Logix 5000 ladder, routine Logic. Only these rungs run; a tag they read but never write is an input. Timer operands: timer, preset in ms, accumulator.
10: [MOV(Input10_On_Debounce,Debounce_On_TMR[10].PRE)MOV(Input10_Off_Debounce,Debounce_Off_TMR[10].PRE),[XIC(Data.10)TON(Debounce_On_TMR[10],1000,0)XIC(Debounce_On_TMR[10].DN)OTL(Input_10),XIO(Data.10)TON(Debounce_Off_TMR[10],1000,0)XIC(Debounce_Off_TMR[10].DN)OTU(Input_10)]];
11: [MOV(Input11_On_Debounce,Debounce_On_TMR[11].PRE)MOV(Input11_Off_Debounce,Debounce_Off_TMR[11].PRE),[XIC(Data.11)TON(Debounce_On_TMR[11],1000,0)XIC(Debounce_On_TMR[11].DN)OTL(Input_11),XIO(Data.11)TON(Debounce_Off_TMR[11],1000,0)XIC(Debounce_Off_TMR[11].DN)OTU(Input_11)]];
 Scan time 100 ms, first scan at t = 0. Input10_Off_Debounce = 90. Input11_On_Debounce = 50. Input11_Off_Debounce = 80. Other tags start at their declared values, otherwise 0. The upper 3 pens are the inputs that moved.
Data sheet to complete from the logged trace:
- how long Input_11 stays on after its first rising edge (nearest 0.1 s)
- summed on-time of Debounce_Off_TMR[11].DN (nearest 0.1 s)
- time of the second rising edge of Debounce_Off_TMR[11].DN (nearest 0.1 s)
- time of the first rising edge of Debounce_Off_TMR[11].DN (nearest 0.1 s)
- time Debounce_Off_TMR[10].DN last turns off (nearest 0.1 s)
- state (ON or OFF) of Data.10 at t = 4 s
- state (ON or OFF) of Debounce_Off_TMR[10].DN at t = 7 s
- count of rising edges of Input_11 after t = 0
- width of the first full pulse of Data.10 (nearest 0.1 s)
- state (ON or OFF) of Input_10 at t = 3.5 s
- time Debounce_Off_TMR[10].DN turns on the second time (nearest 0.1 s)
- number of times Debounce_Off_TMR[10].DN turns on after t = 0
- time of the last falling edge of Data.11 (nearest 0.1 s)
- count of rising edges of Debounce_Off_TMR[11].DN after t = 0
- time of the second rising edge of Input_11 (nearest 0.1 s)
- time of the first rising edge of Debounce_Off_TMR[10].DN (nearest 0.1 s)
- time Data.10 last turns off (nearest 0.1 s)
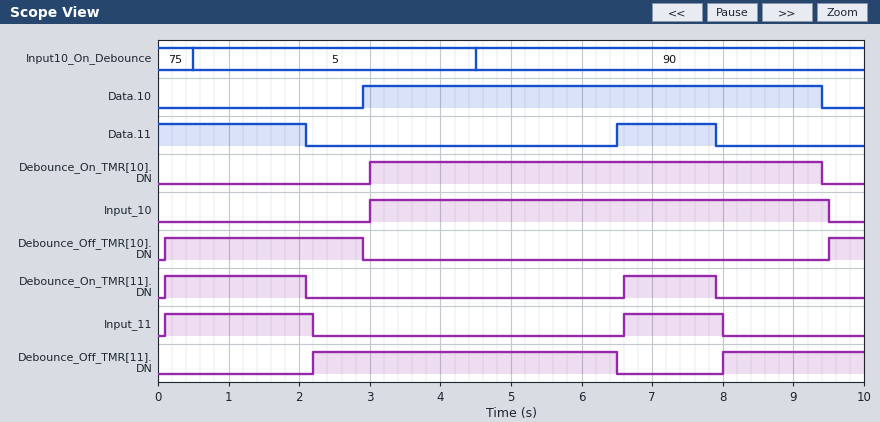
2.1 s
6.3 s
8.0 s
2.2 s
2.9 s
ON
OFF
2
6.5 s
ON
9.5 s
2
7.9 s
2
6.6 s
0.1 s
9.4 s
